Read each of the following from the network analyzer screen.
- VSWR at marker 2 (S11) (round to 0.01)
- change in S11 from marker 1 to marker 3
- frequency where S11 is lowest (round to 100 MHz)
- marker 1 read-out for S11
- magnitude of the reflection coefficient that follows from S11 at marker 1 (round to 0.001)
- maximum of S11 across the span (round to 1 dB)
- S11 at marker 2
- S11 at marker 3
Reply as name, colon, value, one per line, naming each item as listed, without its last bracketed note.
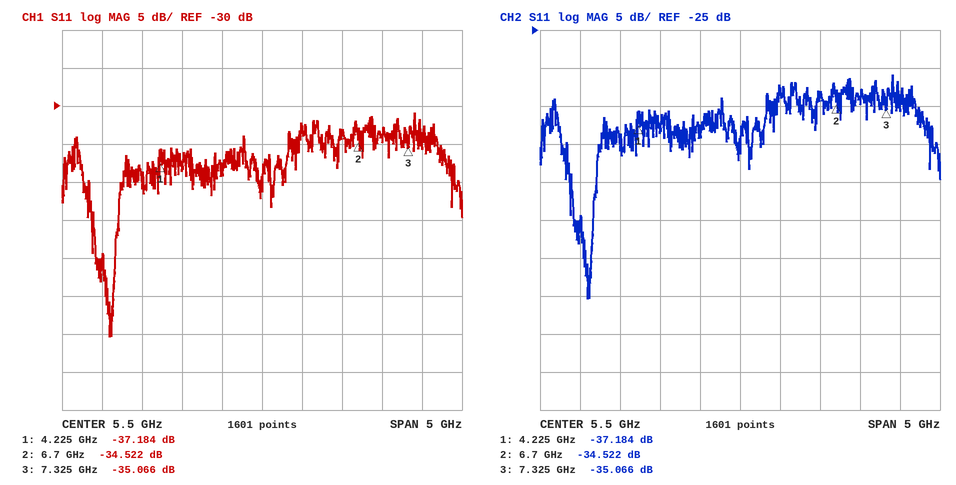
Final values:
VSWR at marker 2 (S11): 1.04
change in S11 from marker 1 to marker 3: 2.118 dB
frequency where S11 is lowest: 3.6 GHz
marker 1 read-out for S11: -37.184 dB
magnitude of the reflection coefficient that follows from S11 at marker 1: 0.014
maximum of S11 across the span: -31 dB
S11 at marker 2: -34.522 dB
S11 at marker 3: -35.066 dB
